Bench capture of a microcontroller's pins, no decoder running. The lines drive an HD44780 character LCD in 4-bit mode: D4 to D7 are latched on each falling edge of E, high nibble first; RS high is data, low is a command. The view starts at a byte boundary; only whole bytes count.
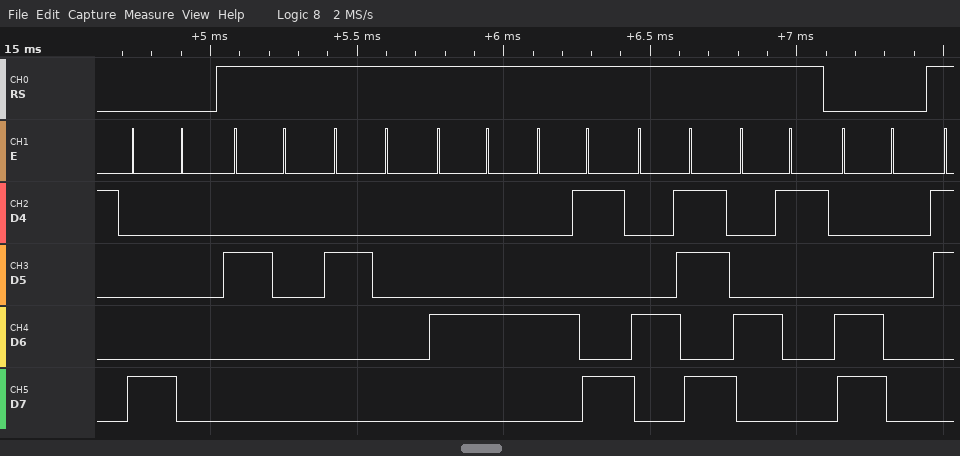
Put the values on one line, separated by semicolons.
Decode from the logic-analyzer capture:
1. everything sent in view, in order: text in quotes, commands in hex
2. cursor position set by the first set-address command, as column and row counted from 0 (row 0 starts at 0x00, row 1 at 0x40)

0x80 "  DIKA" 0xC0; column 0, row 0
